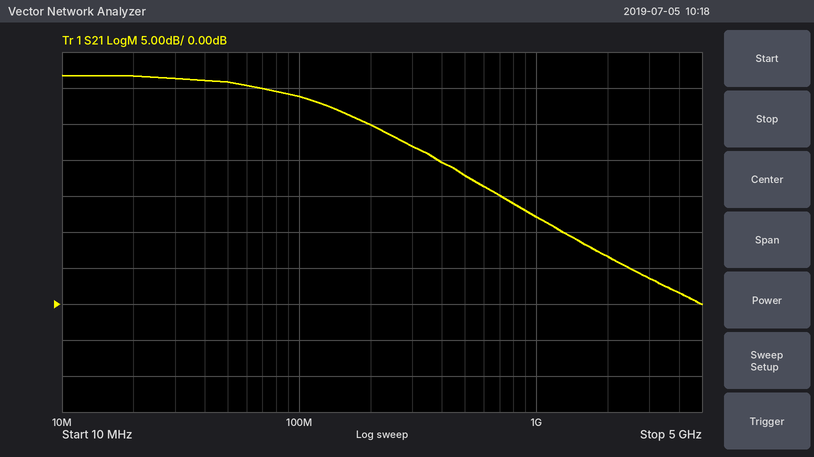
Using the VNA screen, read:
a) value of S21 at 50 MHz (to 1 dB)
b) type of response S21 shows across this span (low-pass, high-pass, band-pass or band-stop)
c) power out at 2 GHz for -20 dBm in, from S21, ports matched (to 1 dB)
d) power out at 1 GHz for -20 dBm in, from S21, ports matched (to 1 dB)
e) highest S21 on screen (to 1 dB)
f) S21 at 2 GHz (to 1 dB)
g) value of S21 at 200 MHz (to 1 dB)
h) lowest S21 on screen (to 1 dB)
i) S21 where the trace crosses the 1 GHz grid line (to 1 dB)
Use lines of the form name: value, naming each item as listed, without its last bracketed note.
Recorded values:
value of S21 at 50 MHz: 31 dB
type of response S21 shows across this span: low-pass
power out at 2 GHz for -20 dBm in, from S21, ports matched: -13 dBm
power out at 1 GHz for -20 dBm in, from S21, ports matched: -8 dBm
highest S21 on screen: 32 dB
S21 at 2 GHz: 7 dB
value of S21 at 200 MHz: 25 dB
lowest S21 on screen: 0 dB
S21 where the trace crosses the 1 GHz grid line: 12 dB
